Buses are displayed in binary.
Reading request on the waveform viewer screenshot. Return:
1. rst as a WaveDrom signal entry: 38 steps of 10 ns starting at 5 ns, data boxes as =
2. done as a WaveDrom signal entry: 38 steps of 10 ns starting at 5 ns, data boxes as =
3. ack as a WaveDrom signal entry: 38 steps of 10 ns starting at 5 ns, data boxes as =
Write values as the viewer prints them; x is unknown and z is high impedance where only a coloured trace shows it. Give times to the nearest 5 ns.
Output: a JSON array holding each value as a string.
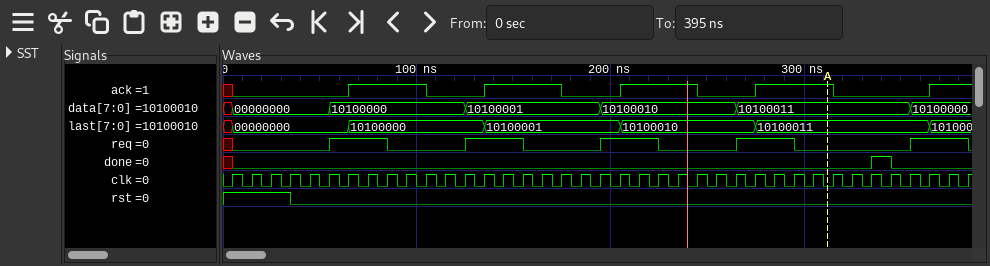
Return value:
["{name: 'rst', wave: '1..0..................................'}", "{name: 'done', wave: '0................................10...'}", "{name: 'ack', wave: '0.....1...0..1...0..1...0..1...0....1.'}"]
